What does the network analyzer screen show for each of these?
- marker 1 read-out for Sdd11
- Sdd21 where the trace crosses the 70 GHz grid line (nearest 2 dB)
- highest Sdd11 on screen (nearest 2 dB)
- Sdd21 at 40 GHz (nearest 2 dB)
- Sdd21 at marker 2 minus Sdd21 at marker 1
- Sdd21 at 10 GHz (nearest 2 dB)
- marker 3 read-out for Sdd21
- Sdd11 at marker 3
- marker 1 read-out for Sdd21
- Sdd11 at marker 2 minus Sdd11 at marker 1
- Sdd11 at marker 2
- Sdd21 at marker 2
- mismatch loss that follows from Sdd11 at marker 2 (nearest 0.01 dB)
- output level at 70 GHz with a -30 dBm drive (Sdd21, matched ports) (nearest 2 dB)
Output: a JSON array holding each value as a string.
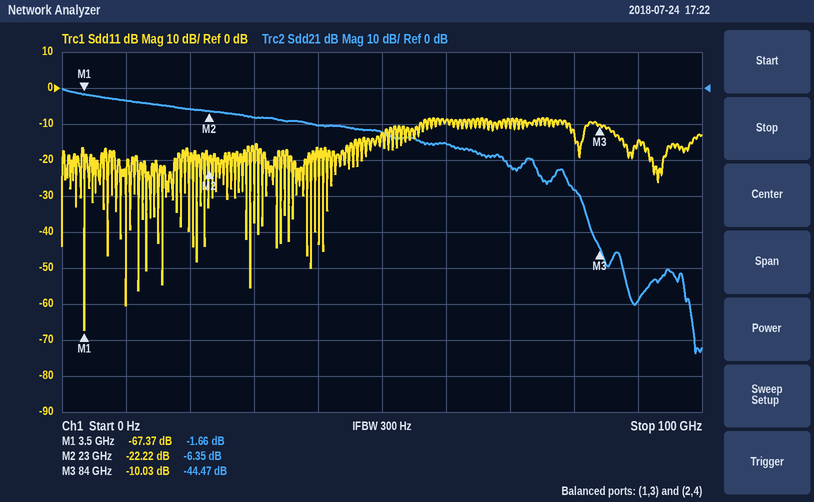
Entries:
["-67.37 dB", "-22 dB", "-8 dB", "-10 dB", "-4.69 dB", "-4 dB", "-44.47 dB", "-10.03 dB", "-1.66 dB", "45.15 dB", "-22.22 dB", "-6.35 dB", "0.03 dB", "-52 dBm"]
